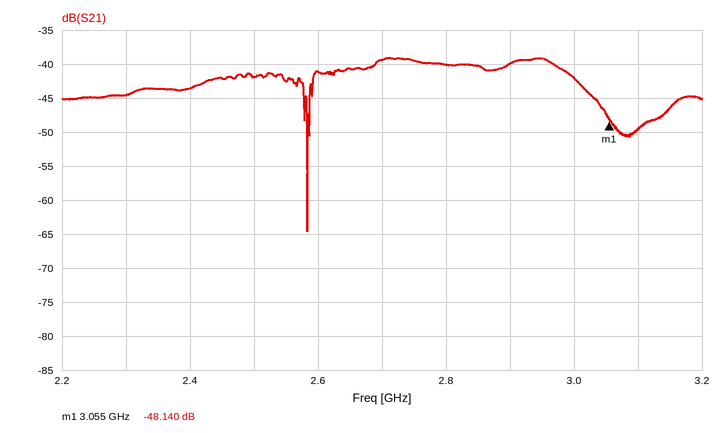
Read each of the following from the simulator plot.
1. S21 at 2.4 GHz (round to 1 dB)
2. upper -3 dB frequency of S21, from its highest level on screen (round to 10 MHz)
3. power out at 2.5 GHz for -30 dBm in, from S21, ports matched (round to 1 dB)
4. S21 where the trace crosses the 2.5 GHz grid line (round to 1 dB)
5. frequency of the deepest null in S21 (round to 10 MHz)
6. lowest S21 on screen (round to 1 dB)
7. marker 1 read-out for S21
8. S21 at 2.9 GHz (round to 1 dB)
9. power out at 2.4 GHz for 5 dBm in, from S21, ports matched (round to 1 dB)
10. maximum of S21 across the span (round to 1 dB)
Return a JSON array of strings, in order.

["-44 dB", "3.00 GHz", "-72 dBm", "-42 dB", "2.58 GHz", "-65 dB", "-48.140 dB", "-40 dB", "-39 dBm", "-39 dB"]
